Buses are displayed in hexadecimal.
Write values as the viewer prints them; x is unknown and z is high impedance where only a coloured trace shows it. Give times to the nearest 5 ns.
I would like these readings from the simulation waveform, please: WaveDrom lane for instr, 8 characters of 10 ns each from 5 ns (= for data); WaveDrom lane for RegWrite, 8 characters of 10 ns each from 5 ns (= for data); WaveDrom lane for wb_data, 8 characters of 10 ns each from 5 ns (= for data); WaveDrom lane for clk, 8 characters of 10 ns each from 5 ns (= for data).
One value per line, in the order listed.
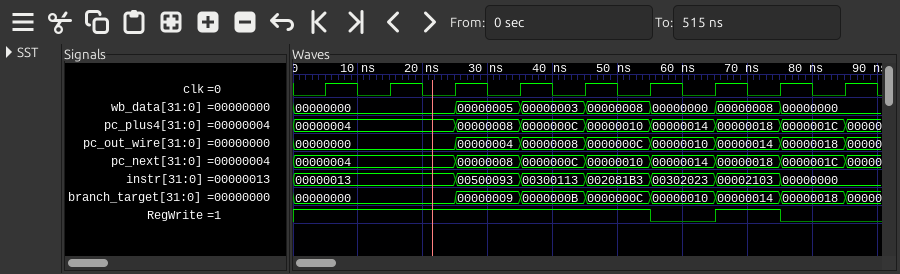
{name: 'instr', wave: '=.======', data: '00000013 00500093 00300113 002081B3 00302023 00002103 00000000'}
{name: 'RegWrite', wave: '1....010'}
{name: 'wb_data', wave: '=.======', data: '00000000 00000005 00000003 00000008 00000000 00000008 00000000'}
{name: 'clk', wave: 'p.......'}
